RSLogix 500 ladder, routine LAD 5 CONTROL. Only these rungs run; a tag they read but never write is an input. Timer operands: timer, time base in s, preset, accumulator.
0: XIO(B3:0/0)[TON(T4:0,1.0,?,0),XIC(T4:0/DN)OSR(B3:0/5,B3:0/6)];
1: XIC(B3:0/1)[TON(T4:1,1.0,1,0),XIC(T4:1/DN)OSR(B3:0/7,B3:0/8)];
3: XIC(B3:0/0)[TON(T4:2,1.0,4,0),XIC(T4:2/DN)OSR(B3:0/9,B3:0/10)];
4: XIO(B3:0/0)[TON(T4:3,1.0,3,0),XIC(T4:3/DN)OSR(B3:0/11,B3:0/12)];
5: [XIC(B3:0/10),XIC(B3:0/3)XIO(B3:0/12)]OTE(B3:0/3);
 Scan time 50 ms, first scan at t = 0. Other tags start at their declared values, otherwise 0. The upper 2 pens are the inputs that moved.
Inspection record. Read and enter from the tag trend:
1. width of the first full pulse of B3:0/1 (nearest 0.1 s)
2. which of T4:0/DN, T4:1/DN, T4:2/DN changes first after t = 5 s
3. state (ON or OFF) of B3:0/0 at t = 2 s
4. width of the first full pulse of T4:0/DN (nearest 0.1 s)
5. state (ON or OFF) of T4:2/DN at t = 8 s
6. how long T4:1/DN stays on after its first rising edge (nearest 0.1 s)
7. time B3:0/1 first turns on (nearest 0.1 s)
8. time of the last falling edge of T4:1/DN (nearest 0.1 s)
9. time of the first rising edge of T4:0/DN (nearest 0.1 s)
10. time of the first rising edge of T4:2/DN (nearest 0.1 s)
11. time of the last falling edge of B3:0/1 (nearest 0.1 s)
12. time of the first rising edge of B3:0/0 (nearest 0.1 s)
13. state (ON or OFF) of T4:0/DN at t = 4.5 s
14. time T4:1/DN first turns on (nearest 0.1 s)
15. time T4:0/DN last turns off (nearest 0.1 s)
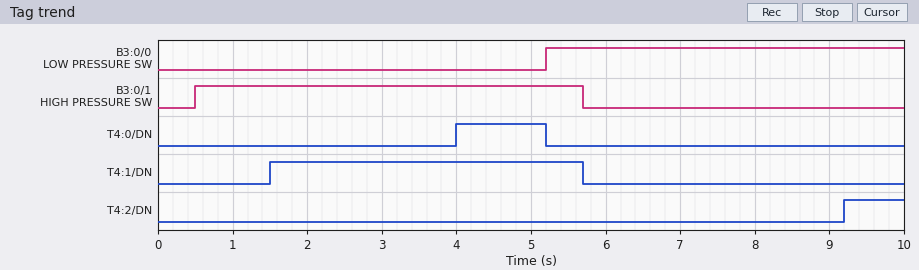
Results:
5.2 s
T4:0/DN
OFF
1.2 s
OFF
4.2 s
0.5 s
5.7 s
4.0 s
9.2 s
5.7 s
5.2 s
ON
1.5 s
5.2 s
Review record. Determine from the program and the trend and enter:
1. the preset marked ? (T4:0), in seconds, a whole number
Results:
4 s
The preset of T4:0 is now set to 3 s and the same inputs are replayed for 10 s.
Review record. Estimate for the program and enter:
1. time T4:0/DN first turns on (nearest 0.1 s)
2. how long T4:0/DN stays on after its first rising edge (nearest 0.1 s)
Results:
3.0 s
2.2 s
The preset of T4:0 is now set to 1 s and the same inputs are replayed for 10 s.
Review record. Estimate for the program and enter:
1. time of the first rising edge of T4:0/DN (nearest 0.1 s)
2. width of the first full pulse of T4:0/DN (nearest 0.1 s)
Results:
1.0 s
4.2 s
